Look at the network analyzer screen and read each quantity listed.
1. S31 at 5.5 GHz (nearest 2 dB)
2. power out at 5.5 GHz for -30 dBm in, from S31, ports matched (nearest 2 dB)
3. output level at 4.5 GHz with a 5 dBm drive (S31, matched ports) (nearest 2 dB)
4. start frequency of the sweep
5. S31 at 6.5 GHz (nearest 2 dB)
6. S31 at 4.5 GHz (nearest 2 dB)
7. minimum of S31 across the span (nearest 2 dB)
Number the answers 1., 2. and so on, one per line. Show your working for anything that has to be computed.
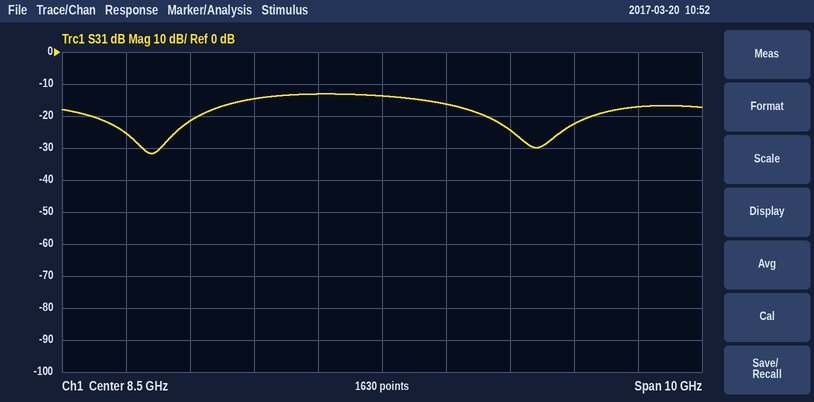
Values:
1. -22 dB
2. -30 dBm + (-22 dB) = -52 dBm
3. 5 dBm + (-26 dB) = -20 dBm
4. 3.5 GHz
5. -14 dB
6. -26 dB
7. -32 dB
